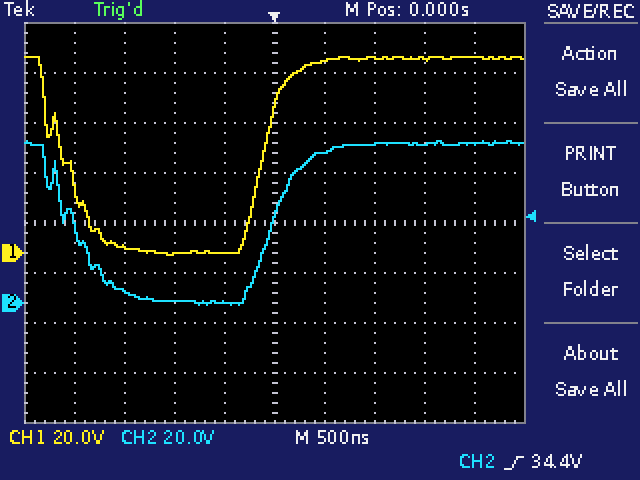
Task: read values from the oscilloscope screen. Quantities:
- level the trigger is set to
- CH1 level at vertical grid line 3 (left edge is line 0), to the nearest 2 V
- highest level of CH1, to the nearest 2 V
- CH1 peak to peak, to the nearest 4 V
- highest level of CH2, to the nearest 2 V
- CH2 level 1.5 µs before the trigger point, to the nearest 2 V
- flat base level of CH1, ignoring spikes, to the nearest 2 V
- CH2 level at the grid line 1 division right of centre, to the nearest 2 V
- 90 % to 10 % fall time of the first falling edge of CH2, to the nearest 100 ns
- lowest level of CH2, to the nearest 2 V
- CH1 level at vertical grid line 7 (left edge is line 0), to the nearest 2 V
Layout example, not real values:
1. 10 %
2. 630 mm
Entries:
1. 34.4 V
2. 0 V
3. 78 V
4. 80 V
5. 64 V
6. 4 V
7. 0 V
8. 60 V
9. 700 ns
10. 0 V
11. 78 V
